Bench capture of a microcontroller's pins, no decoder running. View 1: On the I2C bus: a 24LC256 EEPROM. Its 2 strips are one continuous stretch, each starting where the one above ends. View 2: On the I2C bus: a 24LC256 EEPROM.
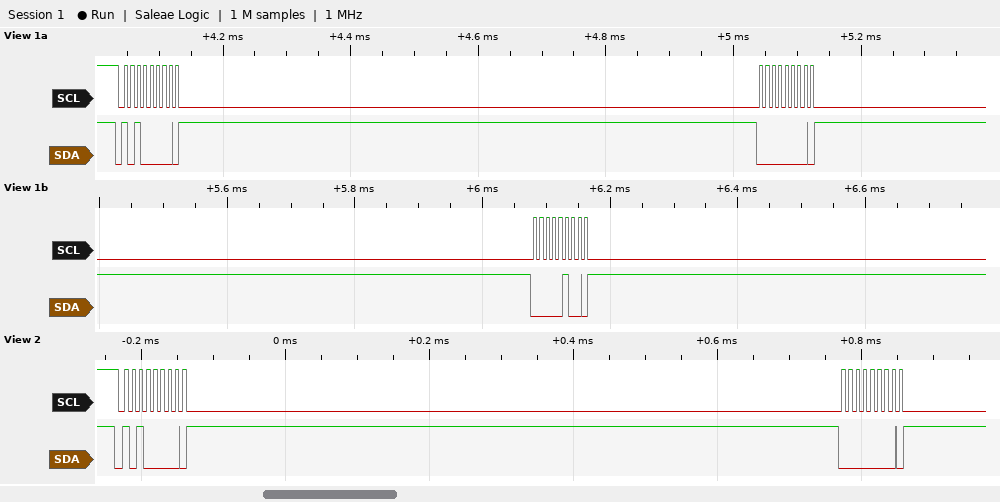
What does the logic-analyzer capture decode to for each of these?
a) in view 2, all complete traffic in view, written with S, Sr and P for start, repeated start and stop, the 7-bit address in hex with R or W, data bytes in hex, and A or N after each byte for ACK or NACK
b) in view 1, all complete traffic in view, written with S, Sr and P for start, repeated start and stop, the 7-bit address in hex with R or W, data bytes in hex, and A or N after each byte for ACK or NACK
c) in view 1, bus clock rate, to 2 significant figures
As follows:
S 50W A 00 A
S 50W A 00 A 04 A
100 kHz
